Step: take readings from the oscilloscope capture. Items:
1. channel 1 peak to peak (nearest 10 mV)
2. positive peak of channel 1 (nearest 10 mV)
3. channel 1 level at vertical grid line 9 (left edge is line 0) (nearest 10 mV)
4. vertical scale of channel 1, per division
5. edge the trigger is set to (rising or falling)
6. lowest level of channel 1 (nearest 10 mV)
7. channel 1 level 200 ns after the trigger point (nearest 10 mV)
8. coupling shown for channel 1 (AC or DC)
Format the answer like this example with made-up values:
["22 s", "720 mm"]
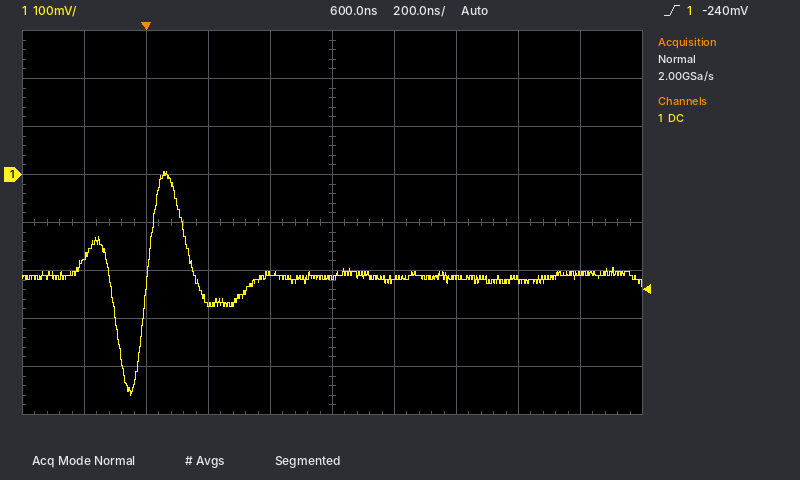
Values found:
["470 mV", "10 mV", "-210 mV", "100 mV", "rising", "-460 mV", "-270 mV", "DC"]
